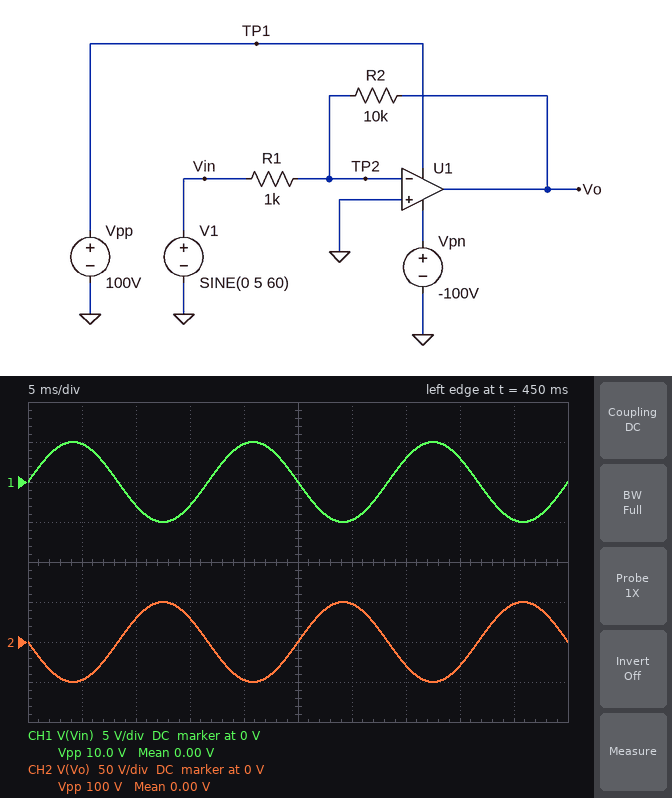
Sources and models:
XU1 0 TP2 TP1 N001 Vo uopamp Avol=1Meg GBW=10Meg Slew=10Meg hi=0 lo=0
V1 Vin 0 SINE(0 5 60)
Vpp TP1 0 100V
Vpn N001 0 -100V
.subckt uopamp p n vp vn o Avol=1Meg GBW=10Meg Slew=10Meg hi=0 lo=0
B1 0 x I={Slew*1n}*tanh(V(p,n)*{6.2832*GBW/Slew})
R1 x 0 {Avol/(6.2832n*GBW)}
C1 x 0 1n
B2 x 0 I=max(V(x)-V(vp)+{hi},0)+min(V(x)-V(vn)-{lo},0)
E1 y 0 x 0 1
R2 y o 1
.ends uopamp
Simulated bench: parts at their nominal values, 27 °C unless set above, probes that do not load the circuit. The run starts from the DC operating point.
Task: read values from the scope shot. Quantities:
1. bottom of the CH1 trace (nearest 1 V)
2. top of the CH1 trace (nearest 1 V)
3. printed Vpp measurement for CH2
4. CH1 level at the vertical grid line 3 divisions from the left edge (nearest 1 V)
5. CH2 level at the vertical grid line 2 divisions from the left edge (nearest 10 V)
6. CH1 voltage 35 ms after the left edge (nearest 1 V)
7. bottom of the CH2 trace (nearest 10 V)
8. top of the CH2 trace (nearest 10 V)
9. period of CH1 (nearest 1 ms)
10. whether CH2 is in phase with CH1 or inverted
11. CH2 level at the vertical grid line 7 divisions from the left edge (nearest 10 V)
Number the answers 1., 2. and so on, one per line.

1. -5 V
2. 5 V
3. 100 V
4. -3 V
5. 30 V
6. 3 V
7. -50 V
8. 50 V
9. 17 ms
10. inverted
11. -30 V
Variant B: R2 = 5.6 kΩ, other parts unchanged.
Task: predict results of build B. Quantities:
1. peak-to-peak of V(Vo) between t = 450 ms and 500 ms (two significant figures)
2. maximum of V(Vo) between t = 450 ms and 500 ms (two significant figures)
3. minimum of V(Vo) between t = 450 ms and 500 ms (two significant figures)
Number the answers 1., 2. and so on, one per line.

1. 56 V
2. 28 V
3. -28 V
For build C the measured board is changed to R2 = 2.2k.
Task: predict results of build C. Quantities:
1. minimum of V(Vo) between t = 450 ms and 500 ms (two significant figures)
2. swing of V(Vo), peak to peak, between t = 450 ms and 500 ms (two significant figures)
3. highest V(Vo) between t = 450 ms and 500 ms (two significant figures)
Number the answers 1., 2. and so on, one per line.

1. -11 V
2. 22 V
3. 11 V
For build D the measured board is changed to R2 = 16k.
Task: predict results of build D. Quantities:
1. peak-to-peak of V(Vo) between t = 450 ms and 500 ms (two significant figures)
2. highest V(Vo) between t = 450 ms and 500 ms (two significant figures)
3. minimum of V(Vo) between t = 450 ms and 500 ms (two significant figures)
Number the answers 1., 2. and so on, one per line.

1. 160 V
2. 80 V
3. -80 V
